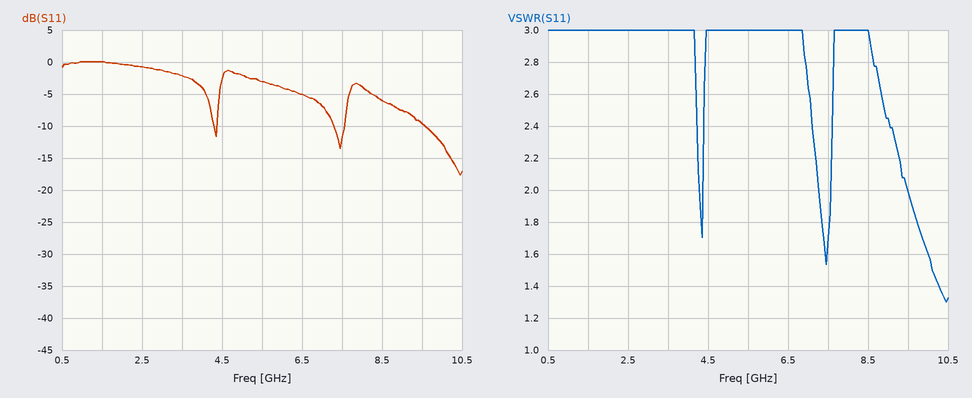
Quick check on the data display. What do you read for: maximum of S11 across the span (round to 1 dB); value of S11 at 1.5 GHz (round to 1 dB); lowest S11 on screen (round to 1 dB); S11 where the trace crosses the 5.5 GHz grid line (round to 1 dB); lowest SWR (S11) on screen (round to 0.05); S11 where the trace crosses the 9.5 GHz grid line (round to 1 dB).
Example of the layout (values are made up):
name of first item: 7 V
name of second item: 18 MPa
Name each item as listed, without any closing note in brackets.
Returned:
maximum of S11 across the span: 0 dB
value of S11 at 1.5 GHz: 0 dB
lowest S11 on screen: -18 dB
S11 where the trace crosses the 5.5 GHz grid line: -3 dB
lowest SWR (S11) on screen: 1.30
S11 where the trace crosses the 9.5 GHz grid line: -10 dB
